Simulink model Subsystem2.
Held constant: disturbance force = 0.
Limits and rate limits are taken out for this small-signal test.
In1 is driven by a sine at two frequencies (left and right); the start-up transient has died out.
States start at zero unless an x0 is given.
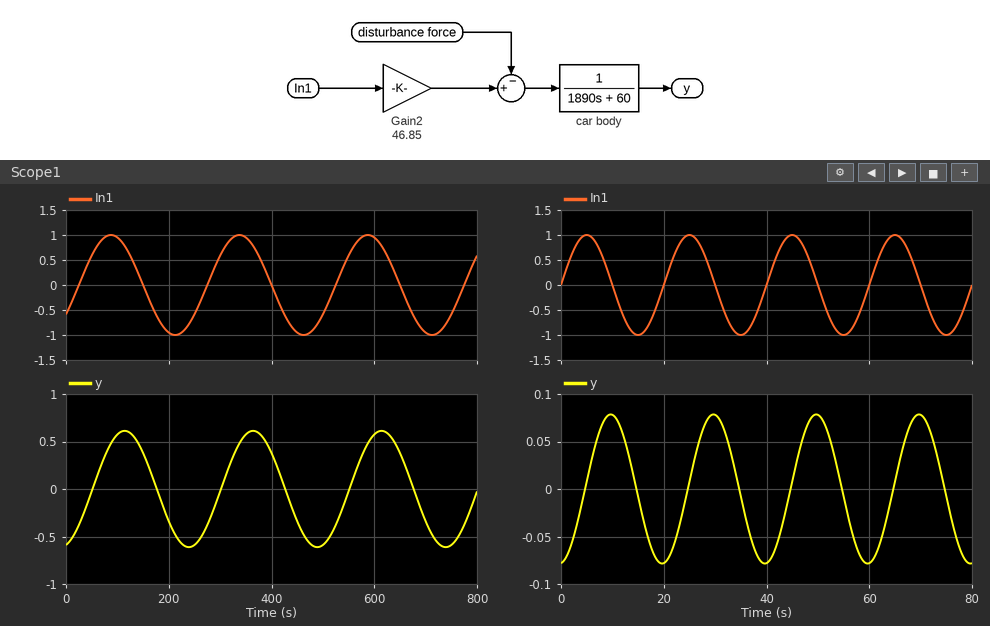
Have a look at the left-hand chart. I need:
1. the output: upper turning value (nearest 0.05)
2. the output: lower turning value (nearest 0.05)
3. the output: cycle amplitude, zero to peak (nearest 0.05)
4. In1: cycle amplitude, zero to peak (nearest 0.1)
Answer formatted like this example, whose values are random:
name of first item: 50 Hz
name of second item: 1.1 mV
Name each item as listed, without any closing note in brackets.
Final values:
the output: upper turning value: 0.60
the output: lower turning value: -0.60
the output: cycle amplitude, zero to peak: 0.60
In1: cycle amplitude, zero to peak: 1.0
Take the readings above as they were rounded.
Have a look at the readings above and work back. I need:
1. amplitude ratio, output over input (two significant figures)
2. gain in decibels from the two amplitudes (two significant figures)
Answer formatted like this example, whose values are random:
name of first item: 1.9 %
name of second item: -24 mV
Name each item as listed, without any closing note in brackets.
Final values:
amplitude ratio, output over input: 0.60
gain in decibels from the two amplitudes: -4.4 dB
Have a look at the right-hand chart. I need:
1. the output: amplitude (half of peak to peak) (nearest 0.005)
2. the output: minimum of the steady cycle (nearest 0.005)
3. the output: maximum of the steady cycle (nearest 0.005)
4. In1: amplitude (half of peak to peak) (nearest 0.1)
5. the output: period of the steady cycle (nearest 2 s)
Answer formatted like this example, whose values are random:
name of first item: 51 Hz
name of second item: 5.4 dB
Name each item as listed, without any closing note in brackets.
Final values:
the output: amplitude (half of peak to peak): 0.080
the output: minimum of the steady cycle: -0.080
the output: maximum of the steady cycle: 0.080
In1: amplitude (half of peak to peak): 1.0
the output: period of the steady cycle: 20 s
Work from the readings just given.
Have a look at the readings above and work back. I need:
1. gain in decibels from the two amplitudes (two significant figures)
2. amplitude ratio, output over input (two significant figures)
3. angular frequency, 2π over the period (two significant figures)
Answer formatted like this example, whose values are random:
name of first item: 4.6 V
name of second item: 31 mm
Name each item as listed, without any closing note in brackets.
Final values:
gain in decibels from the two amplitudes: -22 dB
amplitude ratio, output over input: 0.080
angular frequency, 2π over the period: 0.31 rad/s
